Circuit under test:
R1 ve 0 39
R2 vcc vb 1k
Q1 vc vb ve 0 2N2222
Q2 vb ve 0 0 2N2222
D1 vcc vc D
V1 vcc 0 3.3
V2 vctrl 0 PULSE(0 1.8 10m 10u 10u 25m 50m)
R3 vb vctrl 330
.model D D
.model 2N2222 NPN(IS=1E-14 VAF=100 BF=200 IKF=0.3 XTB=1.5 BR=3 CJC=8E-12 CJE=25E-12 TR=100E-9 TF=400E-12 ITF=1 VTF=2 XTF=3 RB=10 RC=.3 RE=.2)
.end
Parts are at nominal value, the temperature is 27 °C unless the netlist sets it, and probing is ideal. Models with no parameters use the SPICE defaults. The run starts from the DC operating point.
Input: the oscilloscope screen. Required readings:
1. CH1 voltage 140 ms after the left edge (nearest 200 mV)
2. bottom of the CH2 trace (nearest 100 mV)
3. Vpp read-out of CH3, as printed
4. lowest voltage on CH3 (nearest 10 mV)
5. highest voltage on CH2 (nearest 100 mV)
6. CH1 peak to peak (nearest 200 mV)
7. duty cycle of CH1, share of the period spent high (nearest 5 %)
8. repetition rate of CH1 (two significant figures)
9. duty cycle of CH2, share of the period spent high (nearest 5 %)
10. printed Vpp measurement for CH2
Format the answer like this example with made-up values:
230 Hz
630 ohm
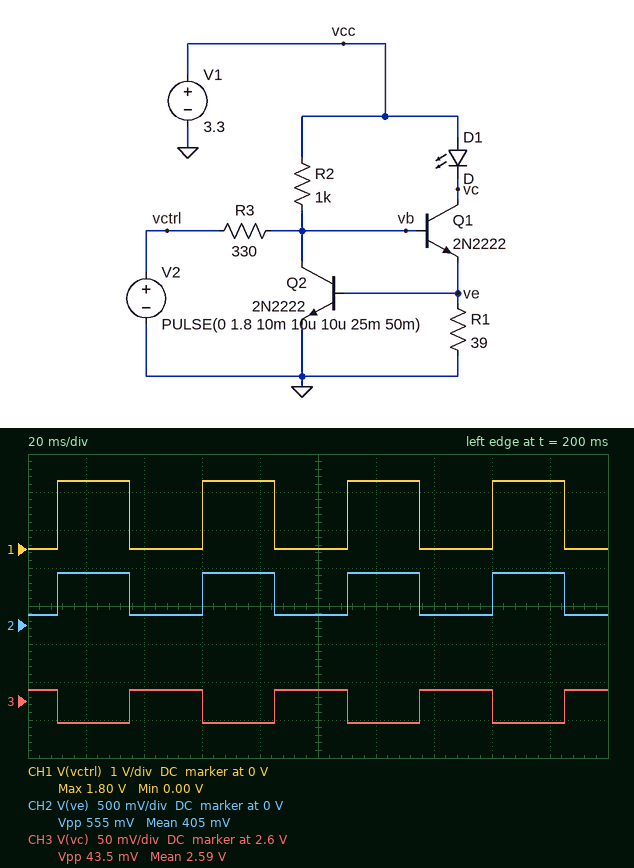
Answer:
0 V
100 mV
43.5 mV
2.57 V
700 mV
1.8 V
50 %
20 Hz
50 %
555 mV
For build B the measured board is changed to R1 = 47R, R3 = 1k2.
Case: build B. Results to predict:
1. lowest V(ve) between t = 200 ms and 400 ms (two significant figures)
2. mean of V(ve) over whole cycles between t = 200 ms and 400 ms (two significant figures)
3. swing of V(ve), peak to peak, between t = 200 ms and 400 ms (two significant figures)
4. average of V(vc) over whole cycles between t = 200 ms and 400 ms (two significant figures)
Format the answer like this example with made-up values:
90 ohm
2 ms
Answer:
650 mV
660 mV
29 mV
2.6 V
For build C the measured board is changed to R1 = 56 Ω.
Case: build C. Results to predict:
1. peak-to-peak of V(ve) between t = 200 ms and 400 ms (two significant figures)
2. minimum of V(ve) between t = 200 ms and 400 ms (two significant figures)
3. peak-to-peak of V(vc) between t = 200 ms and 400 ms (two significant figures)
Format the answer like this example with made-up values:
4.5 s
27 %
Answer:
550 mV
140 mV
42 mV
